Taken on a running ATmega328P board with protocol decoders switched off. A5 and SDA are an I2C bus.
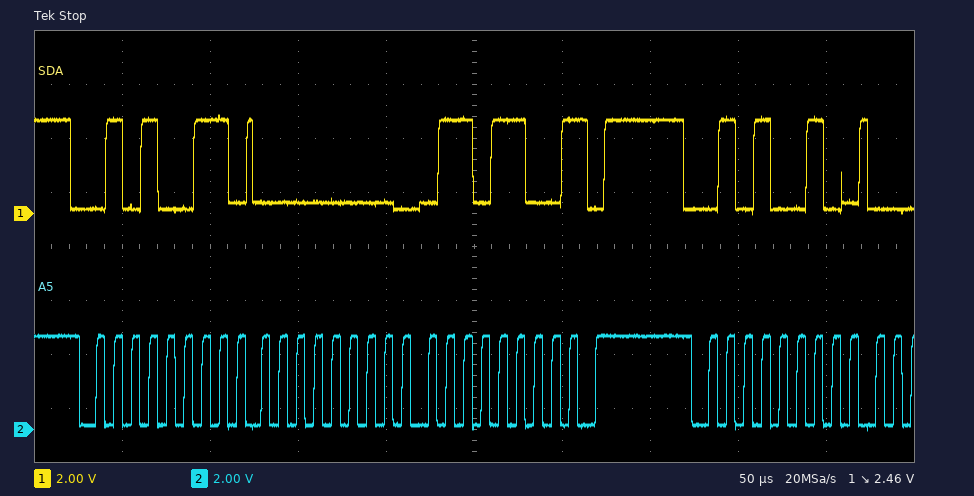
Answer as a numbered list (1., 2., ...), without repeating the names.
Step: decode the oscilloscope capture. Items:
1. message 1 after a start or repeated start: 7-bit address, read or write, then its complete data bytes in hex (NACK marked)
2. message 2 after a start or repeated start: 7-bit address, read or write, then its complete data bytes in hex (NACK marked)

1. 0x29 read: 00 6C NACK
2. 0x29 write
